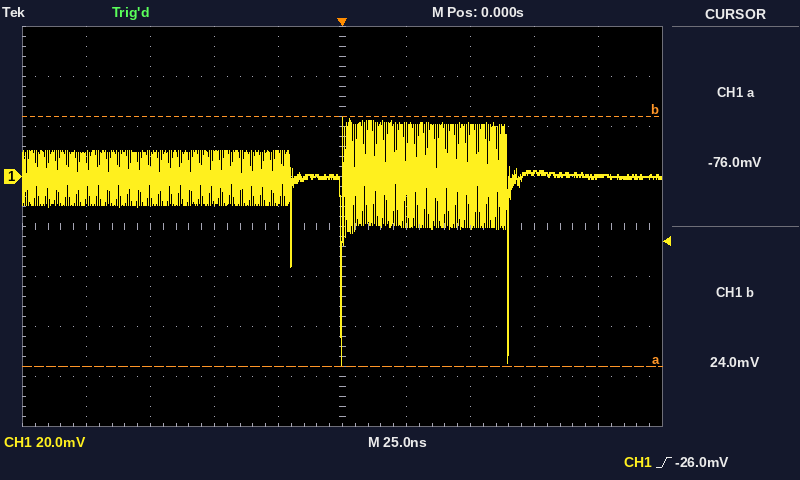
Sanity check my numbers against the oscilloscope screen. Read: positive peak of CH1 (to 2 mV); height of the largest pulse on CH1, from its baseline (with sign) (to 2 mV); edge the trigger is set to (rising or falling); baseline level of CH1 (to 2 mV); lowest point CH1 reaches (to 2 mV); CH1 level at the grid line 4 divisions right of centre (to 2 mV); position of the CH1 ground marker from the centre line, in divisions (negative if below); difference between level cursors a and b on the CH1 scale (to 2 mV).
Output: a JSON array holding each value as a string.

["24 mV", "-76 mV", "rising", "0 mV", "-76 mV", "0 mV", "+1.0 div", "100 mV"]
